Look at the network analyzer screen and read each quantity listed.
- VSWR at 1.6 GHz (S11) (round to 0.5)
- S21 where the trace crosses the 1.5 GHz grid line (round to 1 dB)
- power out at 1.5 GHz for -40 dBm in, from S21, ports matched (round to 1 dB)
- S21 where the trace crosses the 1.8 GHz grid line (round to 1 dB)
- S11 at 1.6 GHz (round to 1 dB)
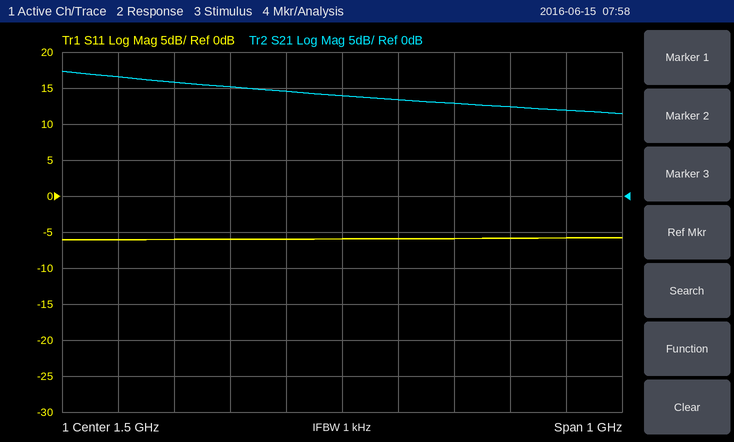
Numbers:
3.0
14 dB
-26 dBm
12 dB
-6 dB
